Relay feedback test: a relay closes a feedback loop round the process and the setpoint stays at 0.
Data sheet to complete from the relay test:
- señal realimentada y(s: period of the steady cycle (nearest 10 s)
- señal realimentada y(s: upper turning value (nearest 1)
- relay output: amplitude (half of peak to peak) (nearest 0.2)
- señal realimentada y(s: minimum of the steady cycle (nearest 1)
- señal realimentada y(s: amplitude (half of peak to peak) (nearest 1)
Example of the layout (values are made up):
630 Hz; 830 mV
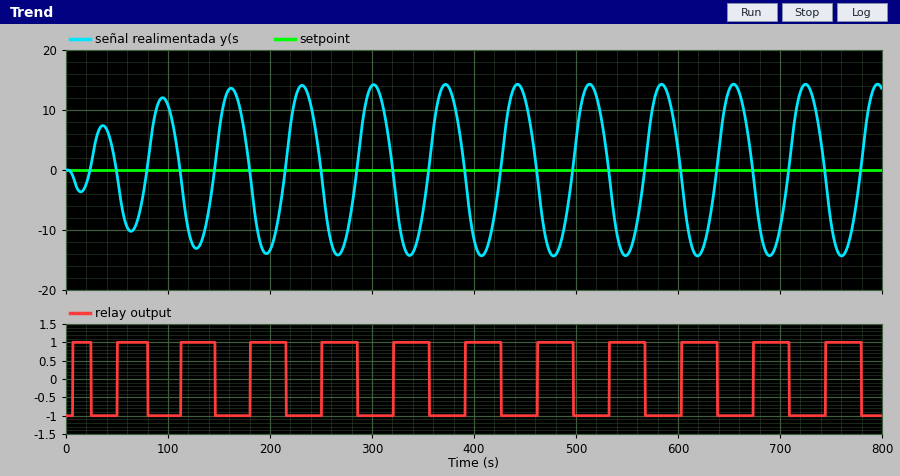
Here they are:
70 s; 14; 1.0; -14; 14
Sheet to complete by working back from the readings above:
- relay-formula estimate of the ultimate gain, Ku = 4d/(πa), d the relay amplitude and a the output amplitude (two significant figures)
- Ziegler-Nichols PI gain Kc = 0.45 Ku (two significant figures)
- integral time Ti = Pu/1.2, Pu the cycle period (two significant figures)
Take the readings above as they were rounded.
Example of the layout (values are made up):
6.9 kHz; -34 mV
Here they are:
0.091; 0.041; 58 s
